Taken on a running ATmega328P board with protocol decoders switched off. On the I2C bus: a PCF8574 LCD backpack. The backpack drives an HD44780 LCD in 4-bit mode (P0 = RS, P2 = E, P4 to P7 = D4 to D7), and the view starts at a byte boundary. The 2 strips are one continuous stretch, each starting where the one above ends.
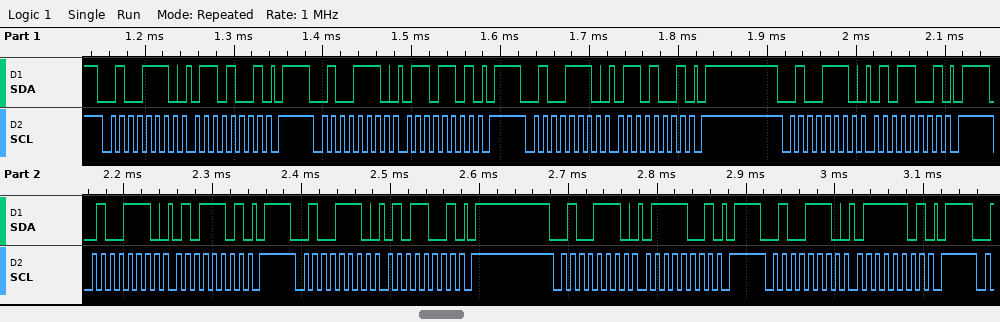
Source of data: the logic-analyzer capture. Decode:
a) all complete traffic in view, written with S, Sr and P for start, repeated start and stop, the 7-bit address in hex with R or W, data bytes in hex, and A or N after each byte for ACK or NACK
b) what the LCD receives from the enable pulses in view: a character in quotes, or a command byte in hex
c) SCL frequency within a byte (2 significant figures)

S 27W A 69 A P S 27W A 6D A P S 27W A 69 A P S 27W A 59 A P S 27W A 5D A P S 27W A 59 A P S 27W A 79 A P S 27W A 7D A P
'e'
100 kHz
